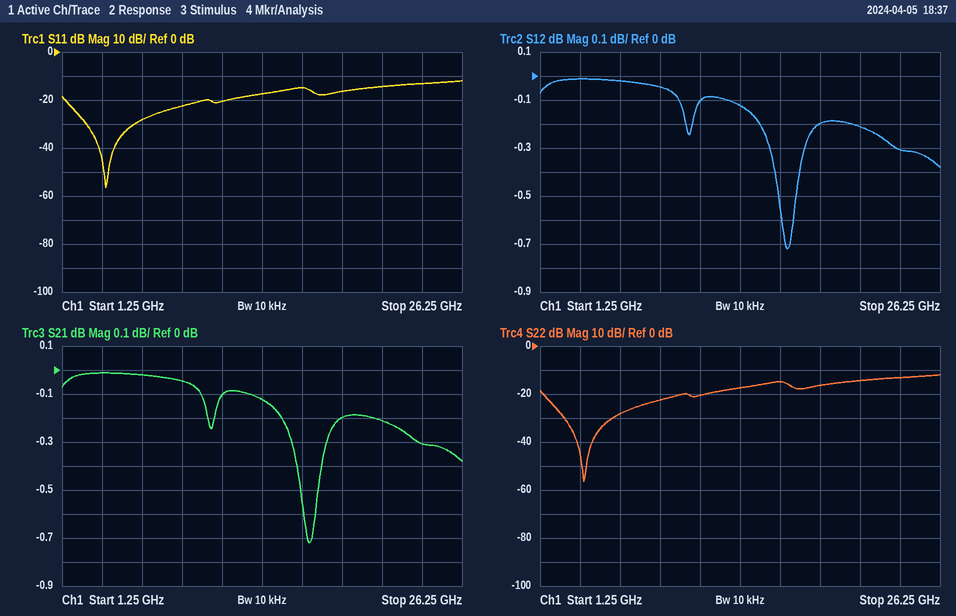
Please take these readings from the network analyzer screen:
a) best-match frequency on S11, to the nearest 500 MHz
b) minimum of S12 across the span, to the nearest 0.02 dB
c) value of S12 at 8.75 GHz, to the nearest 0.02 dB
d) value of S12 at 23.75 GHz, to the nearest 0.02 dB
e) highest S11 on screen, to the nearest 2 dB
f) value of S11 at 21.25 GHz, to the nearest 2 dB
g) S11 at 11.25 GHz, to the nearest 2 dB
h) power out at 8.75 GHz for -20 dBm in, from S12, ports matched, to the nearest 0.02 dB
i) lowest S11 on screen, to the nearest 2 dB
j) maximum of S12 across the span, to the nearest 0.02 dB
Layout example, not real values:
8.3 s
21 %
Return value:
4.0 GHz
-0.72 dB
-0.04 dB
-0.30 dB
-12 dB
-14 dB
-20 dB
-20.04 dBm
-56 dB
-0.02 dB
